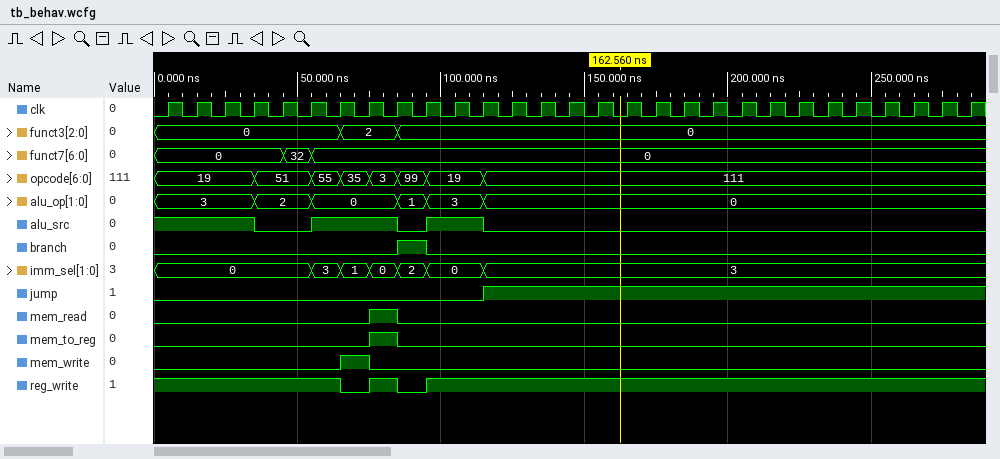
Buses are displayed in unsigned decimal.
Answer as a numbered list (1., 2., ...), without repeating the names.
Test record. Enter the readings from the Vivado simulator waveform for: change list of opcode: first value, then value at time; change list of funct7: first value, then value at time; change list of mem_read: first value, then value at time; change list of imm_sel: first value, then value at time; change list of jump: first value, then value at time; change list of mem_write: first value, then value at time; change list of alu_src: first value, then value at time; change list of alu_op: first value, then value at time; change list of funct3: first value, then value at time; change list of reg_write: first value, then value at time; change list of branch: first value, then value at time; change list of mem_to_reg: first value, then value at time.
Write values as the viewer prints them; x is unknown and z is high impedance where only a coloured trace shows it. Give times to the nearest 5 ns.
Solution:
1. 19, 51 at 35 ns, 55 at 55 ns, 35 at 65 ns, 3 at 75 ns, 99 at 85 ns, 19 at 95 ns, 111 at 115 ns
2. 0, 32 at 45 ns, 0 at 55 ns
3. 0, 1 at 75 ns, 0 at 85 ns
4. 0, 3 at 55 ns, 1 at 65 ns, 0 at 75 ns, 2 at 85 ns, 0 at 95 ns, 3 at 115 ns
5. 0, 1 at 115 ns
6. 0, 1 at 65 ns, 0 at 75 ns
7. 1, 0 at 35 ns, 1 at 55 ns, 0 at 85 ns, 1 at 95 ns, 0 at 115 ns
8. 3, 2 at 35 ns, 0 at 55 ns, 1 at 85 ns, 3 at 95 ns, 0 at 115 ns
9. 0, 2 at 65 ns, 0 at 85 ns
10. 1, 0 at 65 ns, 1 at 75 ns, 0 at 85 ns, 1 at 95 ns
11. 0, 1 at 85 ns, 0 at 95 ns
12. 0, 1 at 75 ns, 0 at 85 ns
